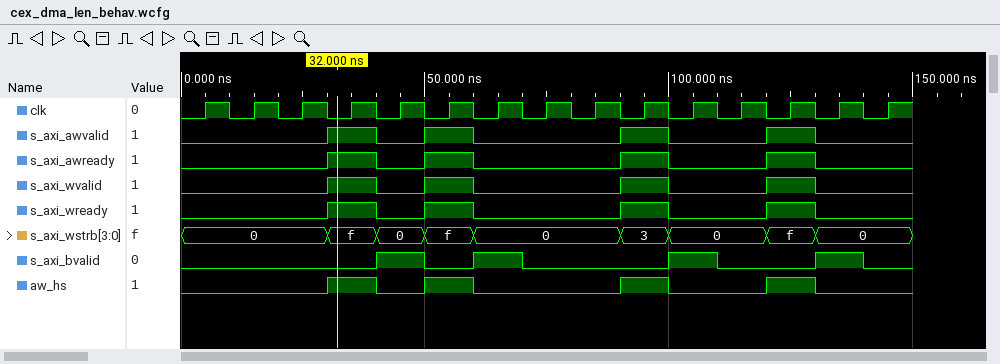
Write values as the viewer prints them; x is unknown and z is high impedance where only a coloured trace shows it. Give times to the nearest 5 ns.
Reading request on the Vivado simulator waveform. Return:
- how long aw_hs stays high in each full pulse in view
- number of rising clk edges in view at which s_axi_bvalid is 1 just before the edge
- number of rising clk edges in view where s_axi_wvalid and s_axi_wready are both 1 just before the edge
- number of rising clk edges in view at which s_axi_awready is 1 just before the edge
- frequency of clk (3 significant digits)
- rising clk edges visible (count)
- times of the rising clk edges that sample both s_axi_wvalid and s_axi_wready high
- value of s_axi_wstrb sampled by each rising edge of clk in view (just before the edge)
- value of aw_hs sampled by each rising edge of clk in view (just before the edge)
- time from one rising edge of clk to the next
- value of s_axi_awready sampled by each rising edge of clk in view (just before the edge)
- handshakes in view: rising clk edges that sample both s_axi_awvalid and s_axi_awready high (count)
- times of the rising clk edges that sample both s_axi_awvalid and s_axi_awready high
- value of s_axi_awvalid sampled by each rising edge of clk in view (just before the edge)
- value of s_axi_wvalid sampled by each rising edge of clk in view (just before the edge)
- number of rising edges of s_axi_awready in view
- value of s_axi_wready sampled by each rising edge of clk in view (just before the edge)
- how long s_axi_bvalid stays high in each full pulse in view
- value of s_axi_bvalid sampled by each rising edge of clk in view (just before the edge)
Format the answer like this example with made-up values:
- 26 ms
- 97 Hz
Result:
- 10 ns, 10 ns, 10 ns, 10 ns
- 4
- 4
- 4
- 100 MHz
- 15
- 35 ns, 55 ns, 95 ns, 125 ns
- 0, 0, 0, f, 0, f, 0, 0, 0, 3, 0, 0, f, 0, 0
- 0 0 0 1 0 1 0 0 0 1 0 0 1 0 0
- 10 ns
- 0 0 0 1 0 1 0 0 0 1 0 0 1 0 0
- 4
- 35 ns, 55 ns, 95 ns, 125 ns
- 0 0 0 1 0 1 0 0 0 1 0 0 1 0 0
- 0 0 0 1 0 1 0 0 0 1 0 0 1 0 0
- 4
- 0 0 0 1 0 1 0 0 0 1 0 0 1 0 0
- 10 ns, 10 ns, 10 ns, 10 ns
- 0 0 0 0 1 0 1 0 0 0 1 0 0 1 0
